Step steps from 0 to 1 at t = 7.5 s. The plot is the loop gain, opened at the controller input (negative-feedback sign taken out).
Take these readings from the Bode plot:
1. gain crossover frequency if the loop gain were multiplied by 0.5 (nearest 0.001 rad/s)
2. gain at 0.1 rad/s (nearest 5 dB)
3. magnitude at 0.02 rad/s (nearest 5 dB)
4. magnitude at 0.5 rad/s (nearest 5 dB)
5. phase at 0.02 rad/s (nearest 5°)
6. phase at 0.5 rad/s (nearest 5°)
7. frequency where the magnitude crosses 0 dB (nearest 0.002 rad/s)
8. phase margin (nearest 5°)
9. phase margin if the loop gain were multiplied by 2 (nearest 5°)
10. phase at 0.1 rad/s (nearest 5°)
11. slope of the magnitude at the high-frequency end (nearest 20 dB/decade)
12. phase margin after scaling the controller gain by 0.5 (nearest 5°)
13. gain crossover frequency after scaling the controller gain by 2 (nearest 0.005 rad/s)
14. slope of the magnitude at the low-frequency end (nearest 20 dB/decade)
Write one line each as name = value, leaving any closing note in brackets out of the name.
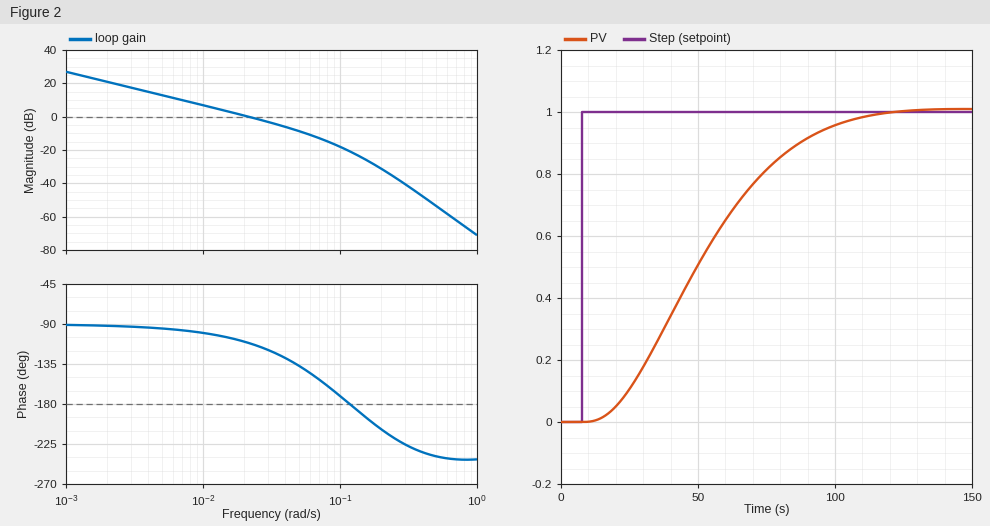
gain crossover frequency if the loop gain were multiplied by 0.5 = 0.011 rad/s
gain at 0.1 rad/s = -20 dB
magnitude at 0.02 rad/s = 0 dB
magnitude at 0.5 rad/s = -55 dB
phase at 0.02 rad/s = -110°
phase at 0.5 rad/s = -240°
frequency where the magnitude crosses 0 dB = 0.022 rad/s
phase margin = 70°
phase margin if the loop gain were multiplied by 2 = 50°
phase at 0.1 rad/s = -170°
slope of the magnitude at the high-frequency end = -60 dB/decade
phase margin after scaling the controller gain by 0.5 = 80°
gain crossover frequency after scaling the controller gain by 2 = 0.040 rad/s
slope of the magnitude at the low-frequency end = -20 dB/decade
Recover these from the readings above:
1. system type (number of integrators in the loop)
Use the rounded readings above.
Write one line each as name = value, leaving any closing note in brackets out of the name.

system type = 1
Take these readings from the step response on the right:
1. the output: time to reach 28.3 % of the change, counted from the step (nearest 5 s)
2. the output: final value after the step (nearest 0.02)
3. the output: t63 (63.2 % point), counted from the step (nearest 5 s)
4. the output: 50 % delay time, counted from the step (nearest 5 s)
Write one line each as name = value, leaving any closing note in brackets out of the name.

the output: time to reach 28.3 % of the change, counted from the step = 30 s
the output: final value after the step = 1.00
the output: t63 (63.2 % point), counted from the step = 50 s
the output: 50 % delay time, counted from the step = 40 s
